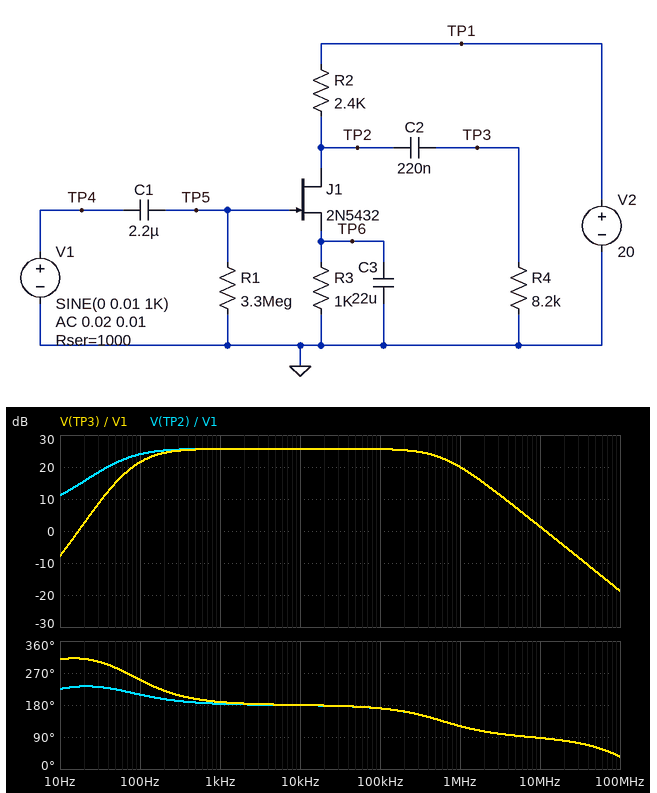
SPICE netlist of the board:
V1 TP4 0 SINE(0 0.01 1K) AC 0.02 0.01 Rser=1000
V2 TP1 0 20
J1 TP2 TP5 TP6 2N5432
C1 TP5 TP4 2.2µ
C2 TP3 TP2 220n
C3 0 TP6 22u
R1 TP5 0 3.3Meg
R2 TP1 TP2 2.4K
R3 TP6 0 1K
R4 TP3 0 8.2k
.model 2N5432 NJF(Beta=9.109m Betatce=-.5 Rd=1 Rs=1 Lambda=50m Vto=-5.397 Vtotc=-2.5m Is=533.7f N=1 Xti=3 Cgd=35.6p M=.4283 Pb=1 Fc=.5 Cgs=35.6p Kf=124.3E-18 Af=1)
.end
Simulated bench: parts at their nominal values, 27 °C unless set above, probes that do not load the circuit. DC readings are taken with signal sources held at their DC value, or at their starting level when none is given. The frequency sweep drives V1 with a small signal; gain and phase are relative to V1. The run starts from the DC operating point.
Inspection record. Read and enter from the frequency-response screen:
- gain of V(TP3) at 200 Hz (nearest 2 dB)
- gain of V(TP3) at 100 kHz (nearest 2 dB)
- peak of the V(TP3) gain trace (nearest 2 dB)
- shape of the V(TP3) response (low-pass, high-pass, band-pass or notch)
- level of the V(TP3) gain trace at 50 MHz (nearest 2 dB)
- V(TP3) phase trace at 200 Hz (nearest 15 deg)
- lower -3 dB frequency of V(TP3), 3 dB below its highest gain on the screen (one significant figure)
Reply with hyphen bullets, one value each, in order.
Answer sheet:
- 24 dB
- 26 dB
- 26 dB
- band-pass
- -12 dB
- 225 deg
- 100 Hz
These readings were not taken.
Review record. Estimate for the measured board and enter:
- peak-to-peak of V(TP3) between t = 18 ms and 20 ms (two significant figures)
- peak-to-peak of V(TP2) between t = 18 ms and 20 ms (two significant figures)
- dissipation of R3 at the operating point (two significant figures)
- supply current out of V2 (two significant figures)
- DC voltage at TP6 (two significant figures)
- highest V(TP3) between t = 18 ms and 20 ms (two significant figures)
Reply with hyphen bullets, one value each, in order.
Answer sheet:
- 380 mV
- 380 mV
- 22 mW
- 4.7 mA
- 4.7 V
- 190 mV
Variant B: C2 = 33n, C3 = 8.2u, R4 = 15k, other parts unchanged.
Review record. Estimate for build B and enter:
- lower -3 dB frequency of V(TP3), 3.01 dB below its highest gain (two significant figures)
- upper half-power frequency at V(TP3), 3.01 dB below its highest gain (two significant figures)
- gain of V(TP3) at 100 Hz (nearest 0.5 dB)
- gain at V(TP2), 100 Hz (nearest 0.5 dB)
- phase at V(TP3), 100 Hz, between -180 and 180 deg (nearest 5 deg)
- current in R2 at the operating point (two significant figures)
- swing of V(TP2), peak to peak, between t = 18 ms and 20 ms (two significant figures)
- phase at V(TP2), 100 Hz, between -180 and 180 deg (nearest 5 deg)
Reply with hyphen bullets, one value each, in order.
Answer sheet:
- 400 Hz
- 570 kHz
- 9.5 dB
- 20.0 dB
- -55 deg
- 4.7 mA
- 410 mV
- -130 deg
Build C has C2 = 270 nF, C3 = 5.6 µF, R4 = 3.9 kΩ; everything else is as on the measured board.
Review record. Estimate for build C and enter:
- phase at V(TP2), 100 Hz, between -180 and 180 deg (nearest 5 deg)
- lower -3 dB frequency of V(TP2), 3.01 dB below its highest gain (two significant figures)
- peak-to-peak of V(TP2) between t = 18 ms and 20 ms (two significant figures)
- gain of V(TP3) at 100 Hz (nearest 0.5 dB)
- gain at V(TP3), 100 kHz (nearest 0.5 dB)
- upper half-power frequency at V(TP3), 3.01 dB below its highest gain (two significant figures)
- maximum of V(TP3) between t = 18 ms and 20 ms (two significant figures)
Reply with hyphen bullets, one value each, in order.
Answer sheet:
- -135 deg
- 320 Hz
- 310 mV
- 10.5 dB
- 24.0 dB
- 710 kHz
- 150 mV
